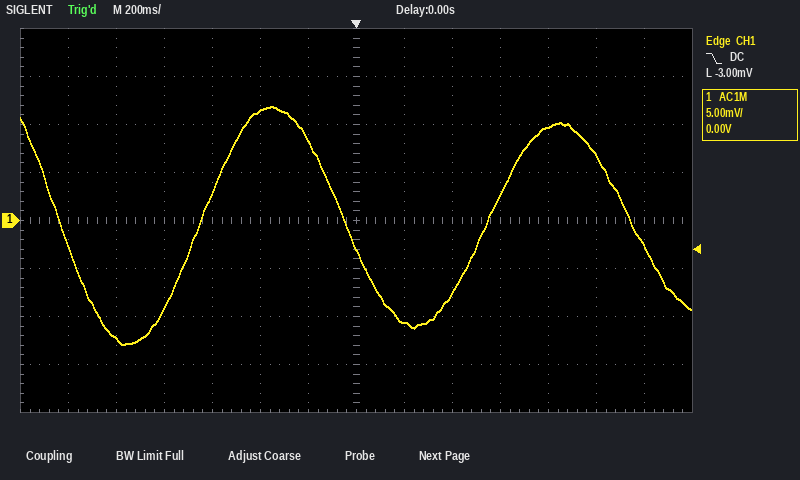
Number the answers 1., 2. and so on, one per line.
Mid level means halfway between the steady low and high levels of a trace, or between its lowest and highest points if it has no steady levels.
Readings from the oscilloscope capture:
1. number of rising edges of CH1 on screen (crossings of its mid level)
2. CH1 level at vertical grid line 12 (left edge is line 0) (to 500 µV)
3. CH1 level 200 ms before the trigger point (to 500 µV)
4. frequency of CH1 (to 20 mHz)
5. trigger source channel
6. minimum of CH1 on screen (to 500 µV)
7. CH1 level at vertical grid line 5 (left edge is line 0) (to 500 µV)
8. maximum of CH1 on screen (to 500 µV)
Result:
1. 2
2. 7.0 mV
3. 8.5 mV
4. 840 mHz
5. CH1
6. -13.0 mV
7. 11.5 mV
8. 12.0 mV
